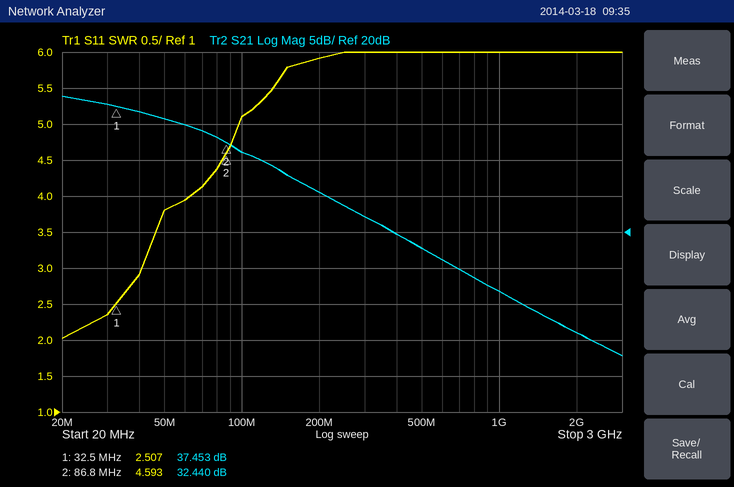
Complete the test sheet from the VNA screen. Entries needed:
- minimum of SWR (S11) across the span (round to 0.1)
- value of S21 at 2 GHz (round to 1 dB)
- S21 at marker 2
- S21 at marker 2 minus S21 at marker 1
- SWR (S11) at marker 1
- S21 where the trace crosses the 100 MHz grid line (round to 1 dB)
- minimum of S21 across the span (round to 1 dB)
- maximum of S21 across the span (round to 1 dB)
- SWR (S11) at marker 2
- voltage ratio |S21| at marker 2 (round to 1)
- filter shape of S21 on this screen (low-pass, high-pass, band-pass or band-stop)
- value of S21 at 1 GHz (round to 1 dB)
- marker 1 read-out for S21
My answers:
2.0
6 dB
32.440 dB
-5.013 dB
2.507
31 dB
3 dB
39 dB
4.593
42
low-pass
12 dB
37.453 dB
